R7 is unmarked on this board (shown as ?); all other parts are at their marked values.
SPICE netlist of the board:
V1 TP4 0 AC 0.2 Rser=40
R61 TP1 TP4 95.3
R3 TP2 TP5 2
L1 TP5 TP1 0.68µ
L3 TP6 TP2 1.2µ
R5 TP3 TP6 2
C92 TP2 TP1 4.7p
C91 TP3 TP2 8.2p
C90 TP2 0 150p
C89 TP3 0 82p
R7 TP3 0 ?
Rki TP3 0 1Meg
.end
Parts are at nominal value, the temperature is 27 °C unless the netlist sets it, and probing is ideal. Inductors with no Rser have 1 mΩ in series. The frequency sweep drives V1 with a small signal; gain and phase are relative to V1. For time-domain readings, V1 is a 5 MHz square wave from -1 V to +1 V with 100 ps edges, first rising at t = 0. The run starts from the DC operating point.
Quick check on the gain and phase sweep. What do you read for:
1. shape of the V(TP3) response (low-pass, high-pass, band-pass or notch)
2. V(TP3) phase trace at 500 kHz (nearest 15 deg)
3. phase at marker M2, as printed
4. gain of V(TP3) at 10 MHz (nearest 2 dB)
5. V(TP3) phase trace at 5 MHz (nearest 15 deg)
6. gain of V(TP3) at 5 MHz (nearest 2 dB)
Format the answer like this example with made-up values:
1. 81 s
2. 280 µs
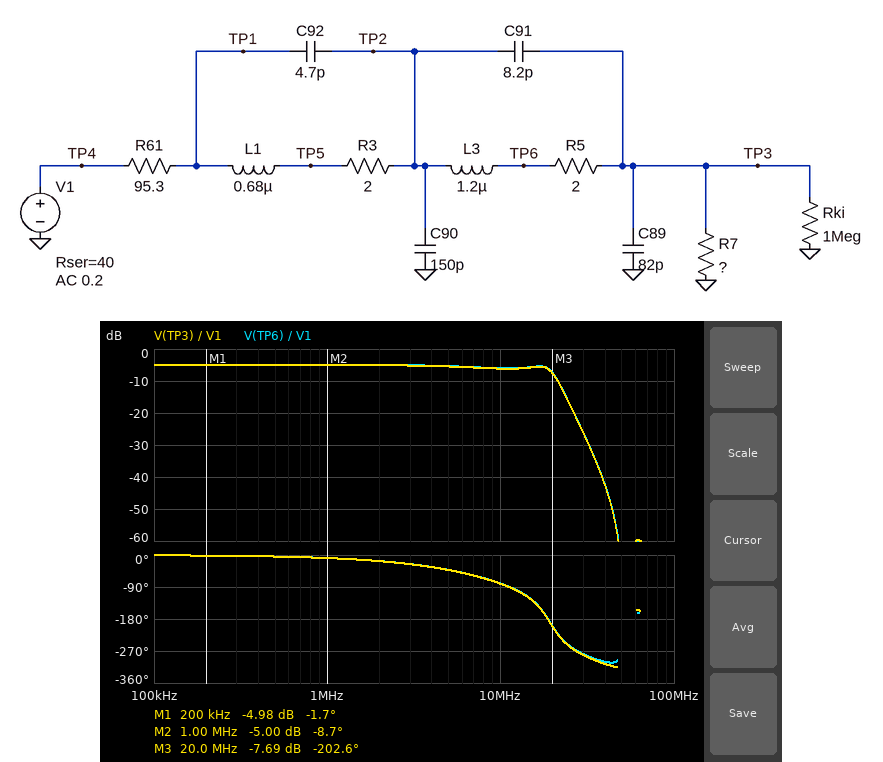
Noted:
1. low-pass
2. 0 deg
3. -8.7 deg
4. -6 dB
5. -45 deg
6. -6 dB
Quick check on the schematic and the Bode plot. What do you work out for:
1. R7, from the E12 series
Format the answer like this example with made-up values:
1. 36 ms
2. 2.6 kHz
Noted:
1. 180 Ω
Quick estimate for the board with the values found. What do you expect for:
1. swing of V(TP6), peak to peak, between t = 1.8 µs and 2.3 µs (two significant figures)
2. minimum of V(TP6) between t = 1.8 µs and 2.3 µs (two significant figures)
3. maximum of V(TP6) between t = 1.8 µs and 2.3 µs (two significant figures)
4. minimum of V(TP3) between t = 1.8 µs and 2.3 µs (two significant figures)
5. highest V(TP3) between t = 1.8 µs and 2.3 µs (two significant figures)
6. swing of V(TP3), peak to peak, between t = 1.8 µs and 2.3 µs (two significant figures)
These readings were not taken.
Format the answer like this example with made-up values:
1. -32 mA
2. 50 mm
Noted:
1. 1.3 V
2. -640 mV
3. 640 mV
4. -640 mV
5. 640 mV
6. 1.3 V
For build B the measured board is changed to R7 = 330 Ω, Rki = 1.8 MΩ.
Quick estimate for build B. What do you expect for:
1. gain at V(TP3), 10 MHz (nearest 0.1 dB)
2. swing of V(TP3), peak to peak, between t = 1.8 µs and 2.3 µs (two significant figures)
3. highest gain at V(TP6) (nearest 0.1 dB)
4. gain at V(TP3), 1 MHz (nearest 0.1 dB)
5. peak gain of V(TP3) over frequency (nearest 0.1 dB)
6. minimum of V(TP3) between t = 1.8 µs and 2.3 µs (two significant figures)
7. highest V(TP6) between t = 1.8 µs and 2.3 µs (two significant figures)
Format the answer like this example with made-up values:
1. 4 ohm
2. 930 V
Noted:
1. -5.0 dB
2. 1.5 V
3. -2.6 dB
4. -3.1 dB
5. -2.7 dB
6. -770 mV
7. 770 mV
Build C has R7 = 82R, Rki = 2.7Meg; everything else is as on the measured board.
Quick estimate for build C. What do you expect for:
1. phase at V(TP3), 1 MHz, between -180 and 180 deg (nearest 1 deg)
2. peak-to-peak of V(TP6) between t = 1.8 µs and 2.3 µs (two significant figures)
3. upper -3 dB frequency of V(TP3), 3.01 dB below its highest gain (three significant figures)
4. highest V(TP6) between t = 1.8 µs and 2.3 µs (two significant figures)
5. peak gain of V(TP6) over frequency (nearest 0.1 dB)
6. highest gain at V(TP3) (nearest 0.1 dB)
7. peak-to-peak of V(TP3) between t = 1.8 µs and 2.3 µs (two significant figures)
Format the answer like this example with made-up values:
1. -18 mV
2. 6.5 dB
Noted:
1. -7 deg
2. 960 mV
3. 18.7 MHz
4. 480 mV
5. -8.3 dB
6. -8.5 dB
7. 940 mV
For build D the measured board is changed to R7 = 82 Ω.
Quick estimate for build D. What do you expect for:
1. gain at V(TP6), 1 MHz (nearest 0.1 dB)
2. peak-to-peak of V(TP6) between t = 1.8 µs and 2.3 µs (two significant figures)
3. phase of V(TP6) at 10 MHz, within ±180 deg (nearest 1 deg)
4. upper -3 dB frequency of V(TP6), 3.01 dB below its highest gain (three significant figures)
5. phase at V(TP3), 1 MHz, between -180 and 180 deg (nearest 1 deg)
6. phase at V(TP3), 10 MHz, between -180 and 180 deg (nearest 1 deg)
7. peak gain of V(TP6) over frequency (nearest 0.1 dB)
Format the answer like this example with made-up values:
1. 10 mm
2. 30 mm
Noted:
1. -8.4 dB
2. 960 mV
3. -77 deg
4. 18.7 MHz
5. -7 deg
6. -78 deg
7. -8.3 dB
